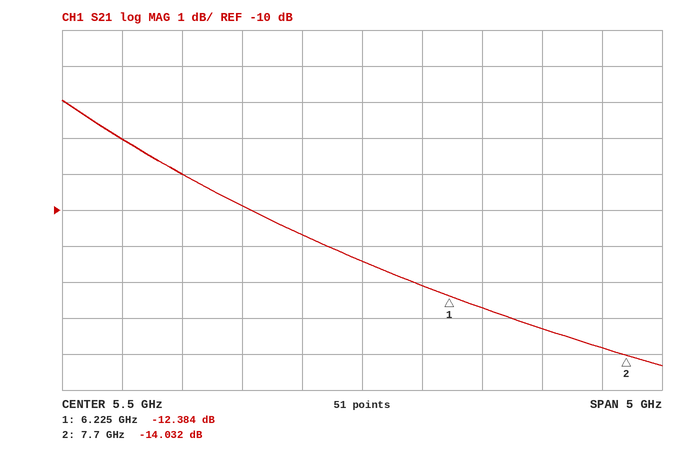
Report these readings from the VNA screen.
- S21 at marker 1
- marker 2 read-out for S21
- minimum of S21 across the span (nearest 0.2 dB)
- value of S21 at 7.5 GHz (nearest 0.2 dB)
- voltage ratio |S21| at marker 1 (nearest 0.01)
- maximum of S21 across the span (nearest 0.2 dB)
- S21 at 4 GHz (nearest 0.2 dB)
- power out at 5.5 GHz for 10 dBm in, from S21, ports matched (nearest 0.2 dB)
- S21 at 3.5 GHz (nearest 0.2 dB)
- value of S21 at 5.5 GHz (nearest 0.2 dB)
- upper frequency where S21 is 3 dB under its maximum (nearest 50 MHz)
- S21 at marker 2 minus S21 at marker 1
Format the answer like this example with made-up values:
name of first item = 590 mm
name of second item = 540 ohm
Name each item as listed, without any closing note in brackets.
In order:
S21 at marker 1 = -12.384 dB
marker 2 read-out for S21 = -14.032 dB
minimum of S21 across the span = -14.4 dB
value of S21 at 7.5 GHz = -13.8 dB
voltage ratio |S21| at marker 1 = 0.24
maximum of S21 across the span = -7.0 dB
S21 at 4 GHz = -9.0 dB
power out at 5.5 GHz for 10 dBm in, from S21, ports matched = -1.4 dBm
S21 at 3.5 GHz = -8.0 dB
value of S21 at 5.5 GHz = -11.4 dB
upper frequency where S21 is 3 dB under its maximum = 4.55 GHz
S21 at marker 2 minus S21 at marker 1 = -1.648 dB
